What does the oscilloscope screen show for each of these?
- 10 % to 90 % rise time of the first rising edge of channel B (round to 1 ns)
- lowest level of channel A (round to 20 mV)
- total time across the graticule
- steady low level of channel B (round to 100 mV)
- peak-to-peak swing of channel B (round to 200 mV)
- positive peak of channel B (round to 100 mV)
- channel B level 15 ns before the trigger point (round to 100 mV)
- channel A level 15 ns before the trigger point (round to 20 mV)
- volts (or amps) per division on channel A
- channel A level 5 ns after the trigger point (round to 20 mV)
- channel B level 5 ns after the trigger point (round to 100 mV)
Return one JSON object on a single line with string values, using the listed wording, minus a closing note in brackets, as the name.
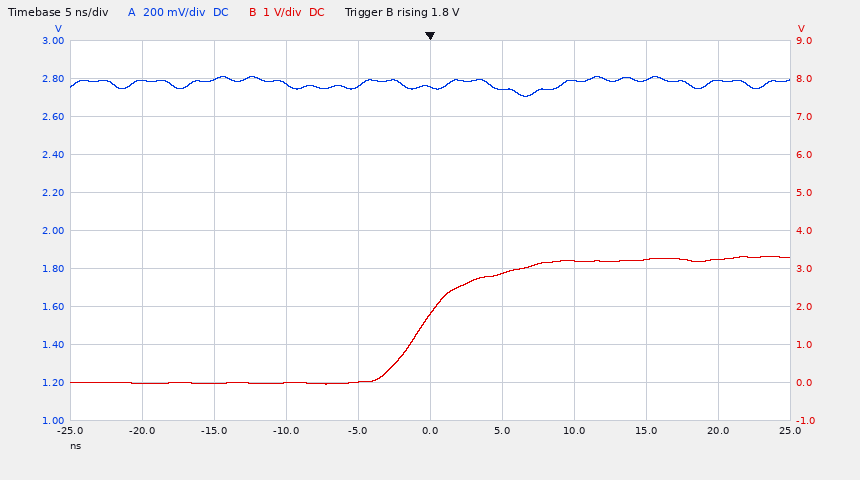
{"10 % to 90 % rise time of the first rising edge of channel B": "8 ns", "lowest level of channel A": "2.70 V", "total time across the graticule": "50 ns", "steady low level of channel B": "0.0 V", "peak-to-peak swing of channel B": "3.4 V", "positive peak of channel B": "3.3 V", "channel B level 15 ns before the trigger point": "0.0 V", "channel A level 15 ns before the trigger point": "2.80 V", "volts (or amps) per division on channel A": "200 mV", "channel A level 5 ns after the trigger point": "2.74 V", "channel B level 5 ns after the trigger point": "2.9 V"}
